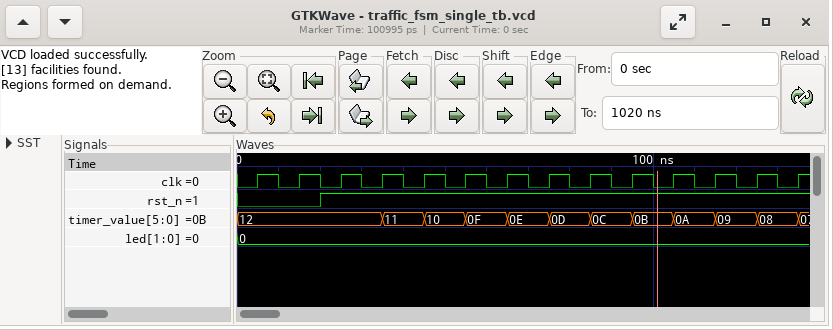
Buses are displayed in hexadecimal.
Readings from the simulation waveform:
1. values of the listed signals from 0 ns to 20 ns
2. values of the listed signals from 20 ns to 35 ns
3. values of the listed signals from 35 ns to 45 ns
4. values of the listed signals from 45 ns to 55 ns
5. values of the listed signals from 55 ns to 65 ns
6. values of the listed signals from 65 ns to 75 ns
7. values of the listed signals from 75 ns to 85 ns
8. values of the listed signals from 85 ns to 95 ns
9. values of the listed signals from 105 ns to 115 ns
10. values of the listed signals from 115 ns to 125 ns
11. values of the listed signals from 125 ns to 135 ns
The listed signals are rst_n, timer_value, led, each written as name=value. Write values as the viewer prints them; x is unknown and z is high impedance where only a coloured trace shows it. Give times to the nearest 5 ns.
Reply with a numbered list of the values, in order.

1. rst_n=0, timer_value=12, led=0
2. rst_n=1, timer_value=12, led=0
3. rst_n=1, timer_value=11, led=0
4. rst_n=1, timer_value=10, led=0
5. rst_n=1, timer_value=0F, led=0
6. rst_n=1, timer_value=0E, led=0
7. rst_n=1, timer_value=0D, led=0
8. rst_n=1, timer_value=0C, led=0
9. rst_n=1, timer_value=0A, led=0
10. rst_n=1, timer_value=09, led=0
11. rst_n=1, timer_value=08, led=0
